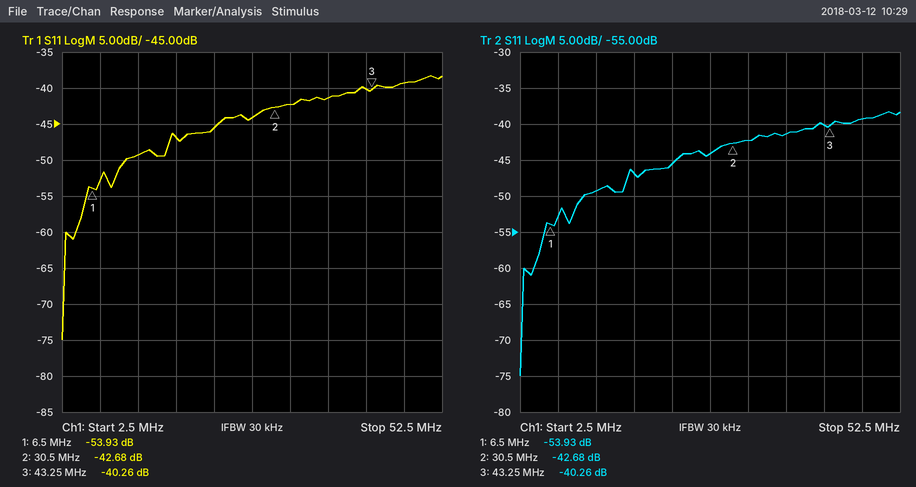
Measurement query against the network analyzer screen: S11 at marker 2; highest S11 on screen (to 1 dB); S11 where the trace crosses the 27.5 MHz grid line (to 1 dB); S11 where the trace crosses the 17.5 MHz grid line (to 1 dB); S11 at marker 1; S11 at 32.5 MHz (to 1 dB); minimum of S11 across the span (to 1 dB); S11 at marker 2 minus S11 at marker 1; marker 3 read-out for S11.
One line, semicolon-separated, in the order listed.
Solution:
-42.68 dB; -38 dB; -44 dB; -47 dB; -53.93 dB; -42 dB; -75 dB; 11.25 dB; -40.26 dB
